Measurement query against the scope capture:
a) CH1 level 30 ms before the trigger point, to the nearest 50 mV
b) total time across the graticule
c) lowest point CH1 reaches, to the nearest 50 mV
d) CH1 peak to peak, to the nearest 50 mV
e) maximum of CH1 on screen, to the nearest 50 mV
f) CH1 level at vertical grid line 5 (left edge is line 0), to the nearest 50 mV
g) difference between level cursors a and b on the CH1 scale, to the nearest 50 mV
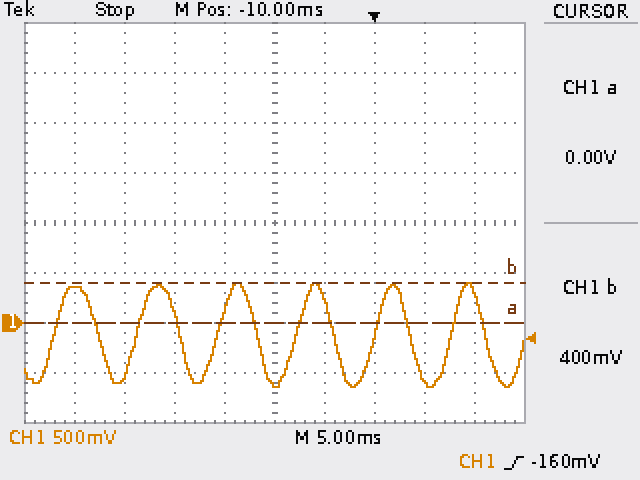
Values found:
350 mV
50 ms
-650 mV
1.05 V
400 mV
-600 mV
400 mV
